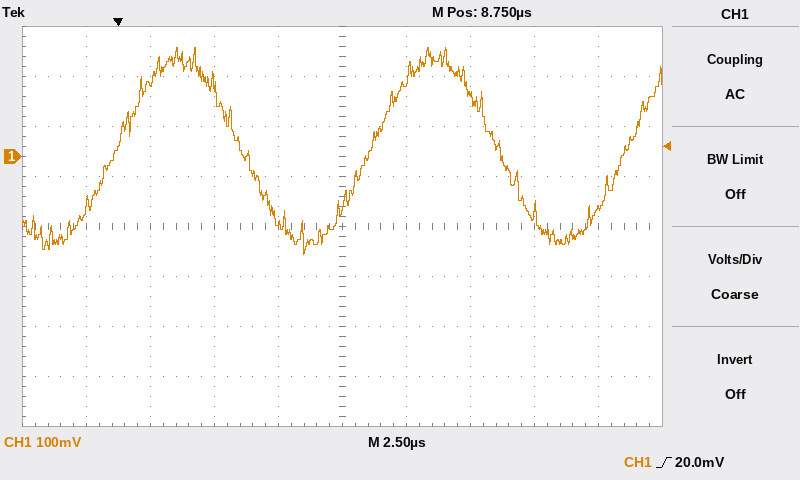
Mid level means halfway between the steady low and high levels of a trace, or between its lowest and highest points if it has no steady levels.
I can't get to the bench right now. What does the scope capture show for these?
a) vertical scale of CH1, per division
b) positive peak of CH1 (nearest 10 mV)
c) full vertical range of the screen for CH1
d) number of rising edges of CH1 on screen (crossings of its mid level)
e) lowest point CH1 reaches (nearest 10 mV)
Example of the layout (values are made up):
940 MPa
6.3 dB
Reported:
100 mV
220 mV
800 mV
3
-200 mV
